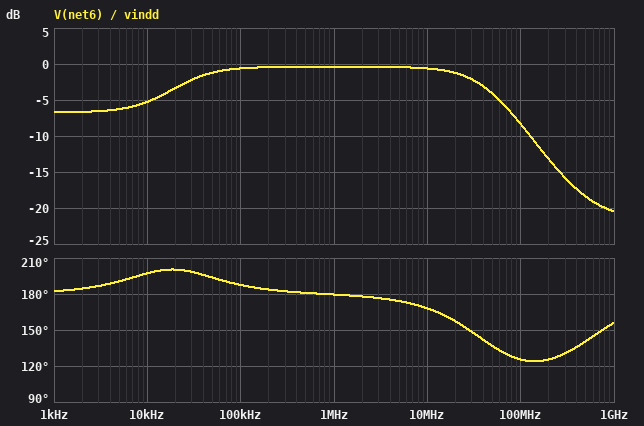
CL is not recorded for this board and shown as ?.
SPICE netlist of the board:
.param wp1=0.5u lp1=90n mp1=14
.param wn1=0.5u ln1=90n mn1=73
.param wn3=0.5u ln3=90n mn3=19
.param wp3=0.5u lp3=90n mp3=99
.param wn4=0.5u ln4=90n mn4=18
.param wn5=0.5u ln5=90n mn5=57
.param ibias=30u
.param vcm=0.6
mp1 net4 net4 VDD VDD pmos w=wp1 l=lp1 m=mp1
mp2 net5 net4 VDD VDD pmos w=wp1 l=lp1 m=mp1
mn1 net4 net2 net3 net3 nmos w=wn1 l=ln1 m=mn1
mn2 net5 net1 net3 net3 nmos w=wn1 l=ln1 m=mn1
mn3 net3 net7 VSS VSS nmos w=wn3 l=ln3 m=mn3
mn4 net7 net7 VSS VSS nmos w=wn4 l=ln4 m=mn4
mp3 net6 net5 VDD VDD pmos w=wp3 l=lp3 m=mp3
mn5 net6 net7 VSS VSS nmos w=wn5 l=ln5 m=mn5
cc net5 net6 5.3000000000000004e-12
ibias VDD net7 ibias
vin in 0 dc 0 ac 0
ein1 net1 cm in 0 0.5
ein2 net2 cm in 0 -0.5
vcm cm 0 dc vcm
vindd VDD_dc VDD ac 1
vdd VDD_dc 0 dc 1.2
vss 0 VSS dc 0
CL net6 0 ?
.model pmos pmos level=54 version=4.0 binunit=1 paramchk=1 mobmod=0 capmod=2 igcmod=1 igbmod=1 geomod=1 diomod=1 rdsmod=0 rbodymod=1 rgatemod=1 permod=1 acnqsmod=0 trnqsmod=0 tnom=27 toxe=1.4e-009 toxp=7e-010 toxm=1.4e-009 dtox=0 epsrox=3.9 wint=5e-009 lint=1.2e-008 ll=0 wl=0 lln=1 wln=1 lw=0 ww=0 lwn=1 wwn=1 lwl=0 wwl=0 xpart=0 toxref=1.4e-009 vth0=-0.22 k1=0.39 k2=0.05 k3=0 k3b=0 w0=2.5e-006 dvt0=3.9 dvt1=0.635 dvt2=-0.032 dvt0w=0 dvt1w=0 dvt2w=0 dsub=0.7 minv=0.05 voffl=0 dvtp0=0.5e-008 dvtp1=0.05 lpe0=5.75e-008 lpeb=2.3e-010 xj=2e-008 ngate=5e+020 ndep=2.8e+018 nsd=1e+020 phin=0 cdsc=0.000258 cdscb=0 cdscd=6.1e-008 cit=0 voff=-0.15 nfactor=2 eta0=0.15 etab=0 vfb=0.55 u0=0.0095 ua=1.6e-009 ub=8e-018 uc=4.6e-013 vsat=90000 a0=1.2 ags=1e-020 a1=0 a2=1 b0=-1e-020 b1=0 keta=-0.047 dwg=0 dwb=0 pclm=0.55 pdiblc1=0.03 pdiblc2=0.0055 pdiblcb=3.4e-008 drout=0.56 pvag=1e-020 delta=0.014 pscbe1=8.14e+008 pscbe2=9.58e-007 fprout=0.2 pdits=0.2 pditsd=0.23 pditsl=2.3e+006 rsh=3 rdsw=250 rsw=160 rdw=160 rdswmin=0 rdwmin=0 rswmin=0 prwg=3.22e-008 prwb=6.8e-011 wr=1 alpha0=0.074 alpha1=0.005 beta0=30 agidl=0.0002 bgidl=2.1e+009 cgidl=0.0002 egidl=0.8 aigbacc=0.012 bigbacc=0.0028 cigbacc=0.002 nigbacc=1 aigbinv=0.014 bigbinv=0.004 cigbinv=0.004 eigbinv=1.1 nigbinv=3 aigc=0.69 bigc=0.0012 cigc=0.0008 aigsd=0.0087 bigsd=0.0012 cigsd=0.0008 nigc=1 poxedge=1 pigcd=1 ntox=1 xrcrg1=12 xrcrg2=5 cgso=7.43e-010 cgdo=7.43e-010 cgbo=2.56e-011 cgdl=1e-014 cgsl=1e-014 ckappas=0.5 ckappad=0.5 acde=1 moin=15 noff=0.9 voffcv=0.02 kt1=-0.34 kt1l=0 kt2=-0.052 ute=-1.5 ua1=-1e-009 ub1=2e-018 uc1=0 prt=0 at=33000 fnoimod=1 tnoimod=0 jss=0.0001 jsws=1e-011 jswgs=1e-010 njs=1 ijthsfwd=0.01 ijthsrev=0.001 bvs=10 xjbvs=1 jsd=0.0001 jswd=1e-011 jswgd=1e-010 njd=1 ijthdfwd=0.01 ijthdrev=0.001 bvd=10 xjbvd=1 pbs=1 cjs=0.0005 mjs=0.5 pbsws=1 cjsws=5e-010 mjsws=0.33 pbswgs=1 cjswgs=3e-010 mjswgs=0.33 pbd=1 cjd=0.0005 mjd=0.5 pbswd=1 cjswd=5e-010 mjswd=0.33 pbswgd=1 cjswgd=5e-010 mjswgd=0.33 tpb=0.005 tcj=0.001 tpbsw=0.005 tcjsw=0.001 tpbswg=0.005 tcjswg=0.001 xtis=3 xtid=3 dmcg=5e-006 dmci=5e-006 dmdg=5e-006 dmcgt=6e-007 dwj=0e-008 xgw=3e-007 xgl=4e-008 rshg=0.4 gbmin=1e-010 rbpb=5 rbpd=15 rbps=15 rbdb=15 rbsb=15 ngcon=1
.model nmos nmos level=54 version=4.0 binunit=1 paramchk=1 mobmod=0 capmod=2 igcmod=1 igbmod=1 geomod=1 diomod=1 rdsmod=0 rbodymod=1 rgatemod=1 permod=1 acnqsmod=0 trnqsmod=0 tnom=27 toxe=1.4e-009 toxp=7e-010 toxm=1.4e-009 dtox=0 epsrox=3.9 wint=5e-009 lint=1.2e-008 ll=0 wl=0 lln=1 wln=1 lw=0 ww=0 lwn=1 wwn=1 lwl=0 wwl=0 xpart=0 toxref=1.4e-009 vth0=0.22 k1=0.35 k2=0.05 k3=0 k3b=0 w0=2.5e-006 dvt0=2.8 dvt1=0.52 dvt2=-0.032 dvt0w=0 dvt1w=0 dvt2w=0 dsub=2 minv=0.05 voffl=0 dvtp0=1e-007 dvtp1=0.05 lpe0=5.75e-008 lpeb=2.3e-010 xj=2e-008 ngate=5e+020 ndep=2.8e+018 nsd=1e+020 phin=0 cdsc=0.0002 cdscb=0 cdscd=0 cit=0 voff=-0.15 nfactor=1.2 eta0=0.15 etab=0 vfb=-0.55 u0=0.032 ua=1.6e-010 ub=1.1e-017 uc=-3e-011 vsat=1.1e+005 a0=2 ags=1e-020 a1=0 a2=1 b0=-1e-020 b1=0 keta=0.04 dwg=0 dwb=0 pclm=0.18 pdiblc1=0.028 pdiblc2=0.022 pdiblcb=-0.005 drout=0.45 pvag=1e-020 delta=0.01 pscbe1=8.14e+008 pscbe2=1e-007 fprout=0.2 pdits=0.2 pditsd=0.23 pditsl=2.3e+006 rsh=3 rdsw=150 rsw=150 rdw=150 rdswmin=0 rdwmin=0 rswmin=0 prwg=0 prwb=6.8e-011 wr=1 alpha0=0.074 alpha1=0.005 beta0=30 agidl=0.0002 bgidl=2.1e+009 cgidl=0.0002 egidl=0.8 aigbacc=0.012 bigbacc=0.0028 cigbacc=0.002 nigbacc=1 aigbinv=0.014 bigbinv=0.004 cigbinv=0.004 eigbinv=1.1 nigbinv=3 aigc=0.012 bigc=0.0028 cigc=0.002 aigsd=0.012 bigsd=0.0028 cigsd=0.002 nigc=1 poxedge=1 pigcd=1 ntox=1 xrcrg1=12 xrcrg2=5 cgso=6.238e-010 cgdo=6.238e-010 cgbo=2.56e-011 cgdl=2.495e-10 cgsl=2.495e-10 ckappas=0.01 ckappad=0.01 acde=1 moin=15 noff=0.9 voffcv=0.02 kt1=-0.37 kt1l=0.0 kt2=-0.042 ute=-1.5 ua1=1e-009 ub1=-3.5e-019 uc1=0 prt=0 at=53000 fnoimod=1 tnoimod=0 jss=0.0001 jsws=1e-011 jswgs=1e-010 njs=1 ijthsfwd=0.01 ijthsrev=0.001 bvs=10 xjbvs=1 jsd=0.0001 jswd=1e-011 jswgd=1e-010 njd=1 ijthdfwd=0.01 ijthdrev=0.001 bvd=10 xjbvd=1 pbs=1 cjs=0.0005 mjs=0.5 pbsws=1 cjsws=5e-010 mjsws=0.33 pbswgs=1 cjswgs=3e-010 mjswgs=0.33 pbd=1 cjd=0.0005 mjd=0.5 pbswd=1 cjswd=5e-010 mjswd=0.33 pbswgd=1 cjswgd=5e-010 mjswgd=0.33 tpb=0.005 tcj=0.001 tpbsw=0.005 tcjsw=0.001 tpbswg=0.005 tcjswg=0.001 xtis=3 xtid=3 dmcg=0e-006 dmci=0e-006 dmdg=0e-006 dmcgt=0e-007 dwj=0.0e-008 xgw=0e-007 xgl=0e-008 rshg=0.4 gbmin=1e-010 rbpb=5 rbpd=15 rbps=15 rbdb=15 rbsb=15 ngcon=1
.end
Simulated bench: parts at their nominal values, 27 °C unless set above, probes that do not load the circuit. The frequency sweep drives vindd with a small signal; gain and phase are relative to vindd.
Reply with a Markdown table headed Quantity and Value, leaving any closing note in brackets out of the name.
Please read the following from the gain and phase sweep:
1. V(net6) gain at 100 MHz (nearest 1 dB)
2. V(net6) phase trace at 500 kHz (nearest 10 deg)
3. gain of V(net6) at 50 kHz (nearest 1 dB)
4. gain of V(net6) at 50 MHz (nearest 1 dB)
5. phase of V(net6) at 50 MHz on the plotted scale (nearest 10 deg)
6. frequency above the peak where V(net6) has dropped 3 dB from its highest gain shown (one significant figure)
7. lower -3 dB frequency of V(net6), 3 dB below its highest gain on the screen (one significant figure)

| Quantity | Value |
|---|---|
| V(net6) gain at 100 MHz | -8 dB |
| V(net6) phase trace at 500 kHz | 180 deg |
| gain of V(net6) at 50 kHz | -1 dB |
| gain of V(net6) at 50 MHz | -4 dB |
| phase of V(net6) at 50 MHz on the plotted scale | 140 deg |
| frequency above the peak where V(net6) has dropped 3 dB from its highest gain shown | 40 MHz |
| lower -3 dB frequency of V(net6), 3 dB below its highest gain on the screen | 20 kHz |
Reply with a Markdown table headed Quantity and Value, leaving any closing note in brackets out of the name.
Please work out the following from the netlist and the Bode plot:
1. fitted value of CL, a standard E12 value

| Quantity | Value |
|---|---|
| fitted value of CL, a standard E12 value | 6.8 pF |
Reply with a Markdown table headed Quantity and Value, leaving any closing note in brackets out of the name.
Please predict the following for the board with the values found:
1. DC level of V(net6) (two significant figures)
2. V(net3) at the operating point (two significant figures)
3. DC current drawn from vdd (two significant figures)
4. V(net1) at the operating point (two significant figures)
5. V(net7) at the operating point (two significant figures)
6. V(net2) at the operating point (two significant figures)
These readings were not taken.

| Quantity | Value |
|---|---|
| DC level of V(net6) | 690 mV |
| V(net3) at the operating point | 350 mV |
| DC current drawn from vdd | 180 µA |
| V(net1) at the operating point | 600 mV |
| V(net7) at the operating point | 350 mV |
| V(net2) at the operating point | 600 mV |
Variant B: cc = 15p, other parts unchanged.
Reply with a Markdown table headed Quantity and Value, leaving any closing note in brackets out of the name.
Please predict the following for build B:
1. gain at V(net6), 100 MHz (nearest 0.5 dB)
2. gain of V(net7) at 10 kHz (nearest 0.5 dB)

| Quantity | Value |
|---|---|
| gain at V(net6), 100 MHz | -8.0 dB |
| gain of V(net7) at 10 kHz | -57.0 dB |
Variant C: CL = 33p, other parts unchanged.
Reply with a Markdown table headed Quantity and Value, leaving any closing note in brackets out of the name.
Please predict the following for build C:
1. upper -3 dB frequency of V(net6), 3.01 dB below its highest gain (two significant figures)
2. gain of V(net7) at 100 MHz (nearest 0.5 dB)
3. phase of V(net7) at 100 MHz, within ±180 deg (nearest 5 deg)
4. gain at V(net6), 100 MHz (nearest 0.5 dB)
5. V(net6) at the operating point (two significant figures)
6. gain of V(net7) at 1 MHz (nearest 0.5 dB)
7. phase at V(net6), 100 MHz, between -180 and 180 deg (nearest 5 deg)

| Quantity | Value |
|---|---|
| upper -3 dB frequency of V(net6), 3.01 dB below its highest gain | 9.9 MHz |
| gain of V(net7) at 100 MHz | -53.0 dB |
| phase of V(net7) at 100 MHz, within ±180 deg | -170 deg |
| gain at V(net6), 100 MHz | -20.5 dB |
| V(net6) at the operating point | 690 mV |
| gain of V(net7) at 1 MHz | -55.5 dB |
| phase at V(net6), 100 MHz, between -180 and 180 deg | 110 deg |
